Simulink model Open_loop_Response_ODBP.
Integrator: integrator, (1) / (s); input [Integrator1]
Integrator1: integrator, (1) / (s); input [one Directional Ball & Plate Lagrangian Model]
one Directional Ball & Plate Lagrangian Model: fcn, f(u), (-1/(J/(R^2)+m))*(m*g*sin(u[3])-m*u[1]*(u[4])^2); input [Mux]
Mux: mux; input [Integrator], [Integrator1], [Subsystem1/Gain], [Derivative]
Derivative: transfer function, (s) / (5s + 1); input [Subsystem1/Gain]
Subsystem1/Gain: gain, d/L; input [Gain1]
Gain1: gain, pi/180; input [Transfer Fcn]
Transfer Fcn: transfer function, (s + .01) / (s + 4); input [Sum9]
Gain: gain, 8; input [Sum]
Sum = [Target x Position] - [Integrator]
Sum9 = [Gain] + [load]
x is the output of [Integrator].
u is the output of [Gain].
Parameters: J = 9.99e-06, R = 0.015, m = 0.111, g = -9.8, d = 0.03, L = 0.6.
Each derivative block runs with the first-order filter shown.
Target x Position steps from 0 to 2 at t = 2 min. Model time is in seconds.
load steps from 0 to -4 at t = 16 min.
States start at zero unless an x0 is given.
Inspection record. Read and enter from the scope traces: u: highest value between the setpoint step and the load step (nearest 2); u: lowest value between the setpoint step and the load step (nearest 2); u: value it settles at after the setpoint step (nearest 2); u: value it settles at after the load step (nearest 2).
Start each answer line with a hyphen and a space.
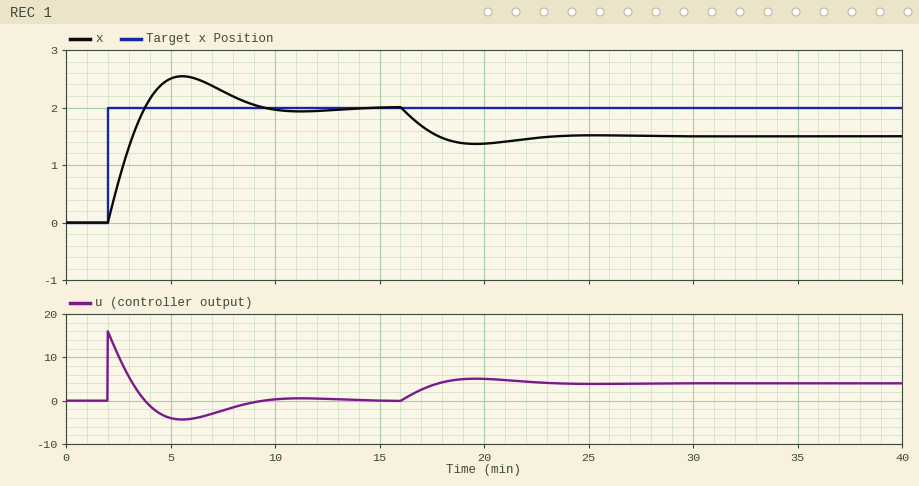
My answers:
- 16
- -4
- 0
- 4
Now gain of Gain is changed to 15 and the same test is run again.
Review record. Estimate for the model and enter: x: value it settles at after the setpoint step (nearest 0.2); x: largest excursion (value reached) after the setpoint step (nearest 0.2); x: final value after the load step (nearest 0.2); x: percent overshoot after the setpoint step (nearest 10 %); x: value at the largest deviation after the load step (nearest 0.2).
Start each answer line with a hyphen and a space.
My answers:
- 2.0
- 2.4
- 1.8
- 20 %
- 1.6
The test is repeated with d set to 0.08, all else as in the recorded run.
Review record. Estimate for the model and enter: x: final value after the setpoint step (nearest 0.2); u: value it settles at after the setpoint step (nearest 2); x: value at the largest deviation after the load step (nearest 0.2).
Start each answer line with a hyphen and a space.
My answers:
- 2.0
- 0
- 1.4
